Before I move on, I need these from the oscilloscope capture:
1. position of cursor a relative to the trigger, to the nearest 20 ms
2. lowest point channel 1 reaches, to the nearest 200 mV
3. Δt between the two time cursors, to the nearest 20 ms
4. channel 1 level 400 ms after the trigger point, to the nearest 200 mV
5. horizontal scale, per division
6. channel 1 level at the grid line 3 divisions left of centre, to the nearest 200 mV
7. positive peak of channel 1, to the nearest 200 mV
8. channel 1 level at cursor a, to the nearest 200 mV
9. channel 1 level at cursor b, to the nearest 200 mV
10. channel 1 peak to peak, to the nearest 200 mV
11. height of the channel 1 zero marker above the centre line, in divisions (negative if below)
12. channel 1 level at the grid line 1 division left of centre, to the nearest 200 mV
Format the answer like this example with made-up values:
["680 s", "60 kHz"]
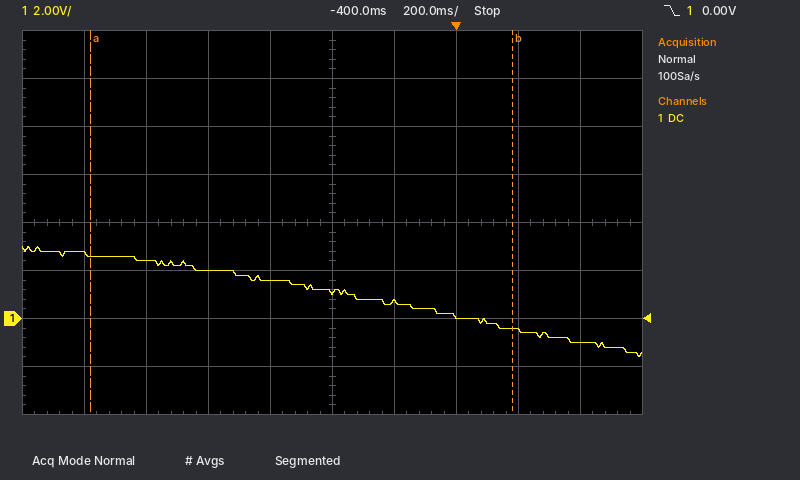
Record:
["-1.18 s", "-1.6 V", "1.36 s", "-1.0 V", "200 ms", "2.4 V", "3.0 V", "2.6 V", "-400 mV", "4.6 V", "-2.0 div", "1.6 V"]
